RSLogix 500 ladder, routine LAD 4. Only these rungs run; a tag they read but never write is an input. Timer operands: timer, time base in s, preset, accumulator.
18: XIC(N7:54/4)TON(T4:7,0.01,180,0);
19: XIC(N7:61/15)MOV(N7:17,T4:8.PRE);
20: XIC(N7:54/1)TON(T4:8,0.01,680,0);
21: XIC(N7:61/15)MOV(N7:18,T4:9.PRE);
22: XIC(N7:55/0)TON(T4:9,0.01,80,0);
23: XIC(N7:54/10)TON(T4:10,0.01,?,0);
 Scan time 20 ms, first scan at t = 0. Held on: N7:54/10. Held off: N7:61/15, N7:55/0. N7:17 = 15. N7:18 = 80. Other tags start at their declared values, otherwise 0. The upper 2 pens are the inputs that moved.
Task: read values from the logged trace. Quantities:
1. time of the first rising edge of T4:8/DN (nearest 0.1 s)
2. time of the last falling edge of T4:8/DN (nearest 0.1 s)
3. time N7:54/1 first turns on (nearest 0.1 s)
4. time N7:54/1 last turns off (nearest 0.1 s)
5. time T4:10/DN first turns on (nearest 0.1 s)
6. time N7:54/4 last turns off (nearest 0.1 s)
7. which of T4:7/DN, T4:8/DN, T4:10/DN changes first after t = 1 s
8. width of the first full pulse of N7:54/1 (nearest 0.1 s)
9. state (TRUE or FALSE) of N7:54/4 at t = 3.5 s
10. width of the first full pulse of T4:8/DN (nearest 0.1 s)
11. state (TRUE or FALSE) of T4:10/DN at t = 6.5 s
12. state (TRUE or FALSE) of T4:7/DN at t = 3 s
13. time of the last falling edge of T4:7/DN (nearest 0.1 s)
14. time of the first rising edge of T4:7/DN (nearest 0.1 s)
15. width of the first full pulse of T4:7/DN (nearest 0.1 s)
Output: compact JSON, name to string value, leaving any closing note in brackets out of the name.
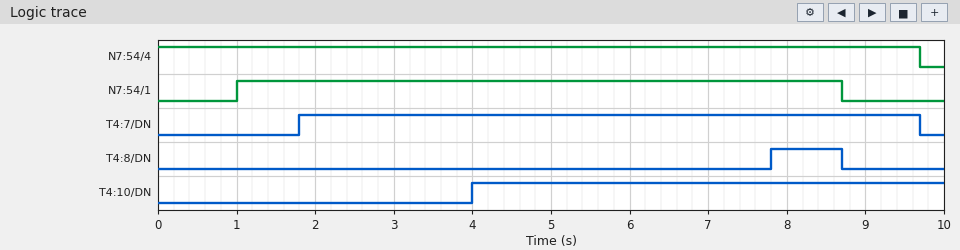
{"time of the first rising edge of T4:8/DN": "7.8 s", "time of the last falling edge of T4:8/DN": "8.7 s", "time N7:54/1 first turns on": "1.0 s", "time N7:54/1 last turns off": "8.7 s", "time T4:10/DN first turns on": "4.0 s", "time N7:54/4 last turns off": "9.7 s", "which of T4:7/DN, T4:8/DN, T4:10/DN changes first after t = 1 s": "T4:7/DN", "width of the first full pulse of N7:54/1": "7.7 s", "state (TRUE or FALSE) of N7:54/4 at t = 3.5 s": "TRUE", "width of the first full pulse of T4:8/DN": "0.9 s", "state (TRUE or FALSE) of T4:10/DN at t = 6.5 s": "TRUE", "state (TRUE or FALSE) of T4:7/DN at t = 3 s": "TRUE", "time of the last falling edge of T4:7/DN": "9.7 s", "time of the first rising edge of T4:7/DN": "1.8 s", "width of the first full pulse of T4:7/DN": "7.9 s"}
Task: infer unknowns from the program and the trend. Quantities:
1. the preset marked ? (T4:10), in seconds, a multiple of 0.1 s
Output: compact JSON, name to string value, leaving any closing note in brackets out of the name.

{"the preset marked ? (T4:10), in seconds, a multiple of 0.1 s": "4.0 s"}
